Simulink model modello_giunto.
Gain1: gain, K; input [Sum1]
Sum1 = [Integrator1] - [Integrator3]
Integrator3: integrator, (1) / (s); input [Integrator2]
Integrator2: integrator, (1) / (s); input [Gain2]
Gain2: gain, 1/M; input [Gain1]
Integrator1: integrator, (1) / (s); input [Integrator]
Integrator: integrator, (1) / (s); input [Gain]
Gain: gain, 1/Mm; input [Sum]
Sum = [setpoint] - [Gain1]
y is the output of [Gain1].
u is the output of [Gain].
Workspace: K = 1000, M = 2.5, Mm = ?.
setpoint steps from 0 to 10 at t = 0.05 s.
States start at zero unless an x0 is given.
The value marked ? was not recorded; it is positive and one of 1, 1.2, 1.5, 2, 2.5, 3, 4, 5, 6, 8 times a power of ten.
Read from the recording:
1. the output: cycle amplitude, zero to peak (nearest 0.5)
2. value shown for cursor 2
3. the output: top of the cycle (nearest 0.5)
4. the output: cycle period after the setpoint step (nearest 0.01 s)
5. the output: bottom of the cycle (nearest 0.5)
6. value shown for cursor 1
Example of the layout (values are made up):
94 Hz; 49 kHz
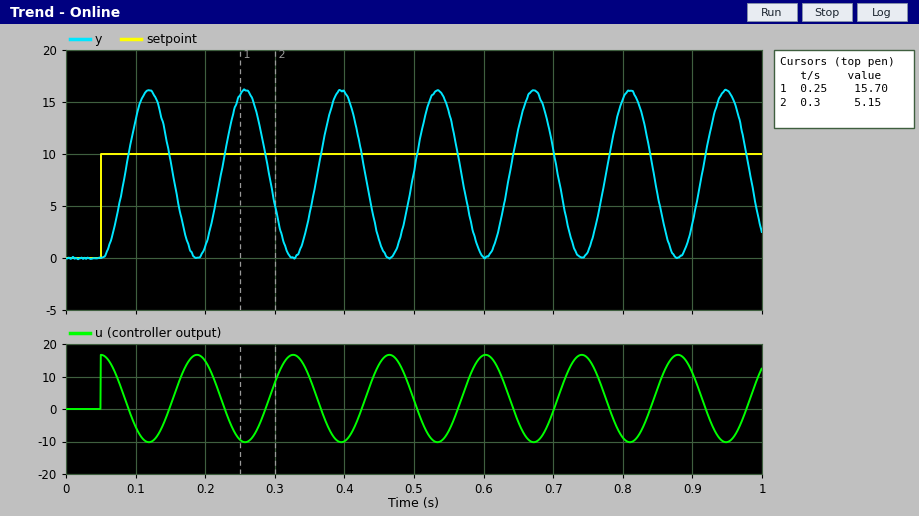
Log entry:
8.0; 5.15; 16.0; 0.14 s; 0.0; 15.70
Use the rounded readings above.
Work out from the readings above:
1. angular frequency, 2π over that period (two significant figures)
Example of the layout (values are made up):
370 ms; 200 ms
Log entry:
45 rad/s
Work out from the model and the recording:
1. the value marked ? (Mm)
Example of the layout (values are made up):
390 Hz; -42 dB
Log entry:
0.6
